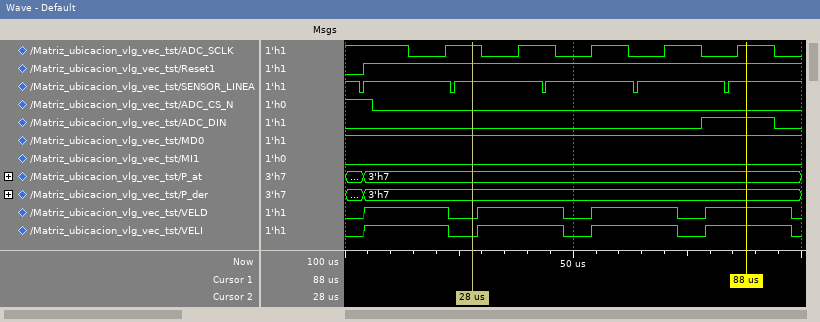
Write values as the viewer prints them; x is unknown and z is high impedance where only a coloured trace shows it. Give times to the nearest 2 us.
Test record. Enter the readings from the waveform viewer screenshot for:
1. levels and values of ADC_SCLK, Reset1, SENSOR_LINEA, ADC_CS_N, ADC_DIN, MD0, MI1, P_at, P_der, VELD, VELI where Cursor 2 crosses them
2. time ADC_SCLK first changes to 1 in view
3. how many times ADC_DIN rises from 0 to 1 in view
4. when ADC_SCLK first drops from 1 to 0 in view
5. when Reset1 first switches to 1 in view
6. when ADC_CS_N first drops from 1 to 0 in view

ADC_SCLK=1, Reset1=1, SENSOR_LINEA=1, ADC_CS_N=0, ADC_DIN=0, MD0=1, MI1=0, P_at=3'h7, P_der=3'h7, VELD=0, VELI=0
22 us
1
14 us
4 us
6 us
